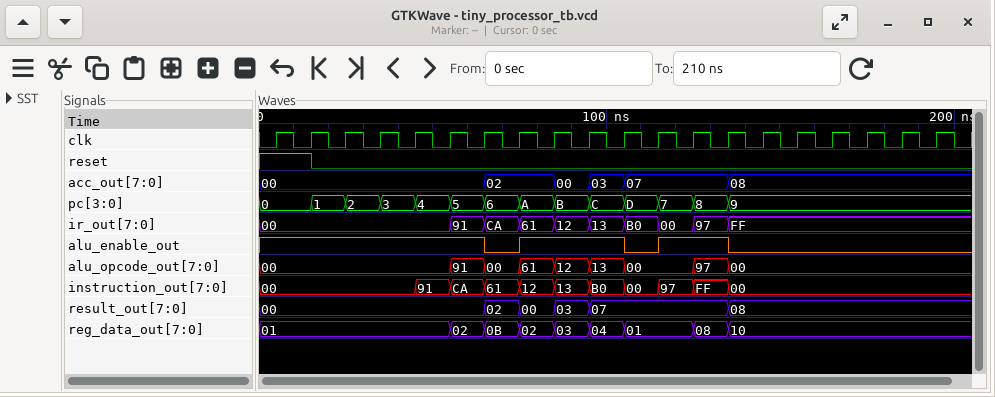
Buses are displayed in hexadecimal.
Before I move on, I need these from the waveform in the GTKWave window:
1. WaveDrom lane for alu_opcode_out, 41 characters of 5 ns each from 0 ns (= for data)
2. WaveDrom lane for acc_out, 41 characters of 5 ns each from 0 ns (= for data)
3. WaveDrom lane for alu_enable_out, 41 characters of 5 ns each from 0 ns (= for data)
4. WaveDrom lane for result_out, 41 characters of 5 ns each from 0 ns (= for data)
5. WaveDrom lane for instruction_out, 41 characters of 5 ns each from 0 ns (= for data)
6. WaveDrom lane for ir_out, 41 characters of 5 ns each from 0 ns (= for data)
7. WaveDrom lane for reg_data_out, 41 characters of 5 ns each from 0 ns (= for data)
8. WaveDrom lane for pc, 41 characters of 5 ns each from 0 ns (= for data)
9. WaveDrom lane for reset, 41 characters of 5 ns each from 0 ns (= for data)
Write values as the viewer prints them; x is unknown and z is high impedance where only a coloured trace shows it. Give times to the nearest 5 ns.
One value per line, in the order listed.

{name: 'alu_opcode_out', wave: '=..........=.=.=.=.=.=...=.=.............', data: '00 91 00 61 12 13 00 97 00'}
{name: 'acc_out', wave: '=............=...=.=.=.....=.............', data: '00 02 00 03 07 08'}
{name: 'alu_enable_out', wave: '1............0.1.....0.1...0.............'}
{name: 'result_out', wave: '=............=.=.=.=.......=.............', data: '00 02 00 03 07 08'}
{name: 'instruction_out', wave: '=........=.=.=.=.=.=.=.=.=.=.............', data: '00 91 CA 61 12 13 B0 00 97 FF 00'}
{name: 'ir_out', wave: '=..........=.=.=.=.=.=.=.=.=.............', data: '00 91 CA 61 12 13 B0 00 97 FF'}
{name: 'reg_data_out', wave: '=..........=.=.=.=.=.=...=.=.............', data: '01 02 0B 02 03 04 01 08 10'}
{name: 'pc', wave: '=..=.=.=.=.=.=.=.=.=.=.=.=.=.............', data: '0 1 2 3 4 5 6 A B C D 7 8 9'}
{name: 'reset', wave: '1..0.....................................'}
